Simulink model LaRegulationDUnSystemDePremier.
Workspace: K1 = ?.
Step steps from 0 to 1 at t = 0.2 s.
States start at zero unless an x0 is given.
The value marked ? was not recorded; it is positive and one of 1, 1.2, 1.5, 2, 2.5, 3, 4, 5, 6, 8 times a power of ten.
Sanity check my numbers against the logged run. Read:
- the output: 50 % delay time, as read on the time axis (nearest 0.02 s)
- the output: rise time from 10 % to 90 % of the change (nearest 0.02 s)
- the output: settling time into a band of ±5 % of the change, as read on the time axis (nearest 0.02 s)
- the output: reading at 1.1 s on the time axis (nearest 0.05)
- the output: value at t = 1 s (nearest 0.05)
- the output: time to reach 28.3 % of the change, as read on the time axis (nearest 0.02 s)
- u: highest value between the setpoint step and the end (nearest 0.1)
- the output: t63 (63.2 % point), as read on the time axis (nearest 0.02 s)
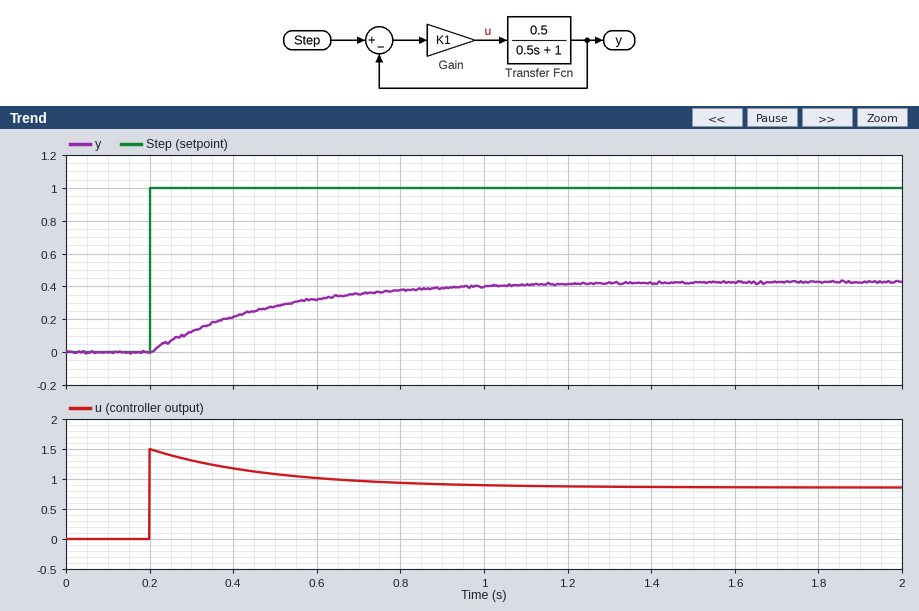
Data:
0.40 s
0.62 s
1.06 s
0.40
0.40
0.30 s
1.5
0.48 s
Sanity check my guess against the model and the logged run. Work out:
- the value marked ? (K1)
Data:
1.5
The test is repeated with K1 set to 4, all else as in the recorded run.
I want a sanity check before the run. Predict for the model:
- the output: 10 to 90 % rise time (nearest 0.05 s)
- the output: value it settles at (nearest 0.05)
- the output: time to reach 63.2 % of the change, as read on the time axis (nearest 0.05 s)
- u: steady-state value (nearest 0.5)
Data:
0.35 s
0.65
0.35 s
1.5
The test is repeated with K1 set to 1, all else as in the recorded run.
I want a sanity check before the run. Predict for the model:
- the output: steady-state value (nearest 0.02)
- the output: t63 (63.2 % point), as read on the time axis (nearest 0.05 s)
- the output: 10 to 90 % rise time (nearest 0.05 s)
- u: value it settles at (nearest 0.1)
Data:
0.34
0.55 s
0.75 s
0.7
